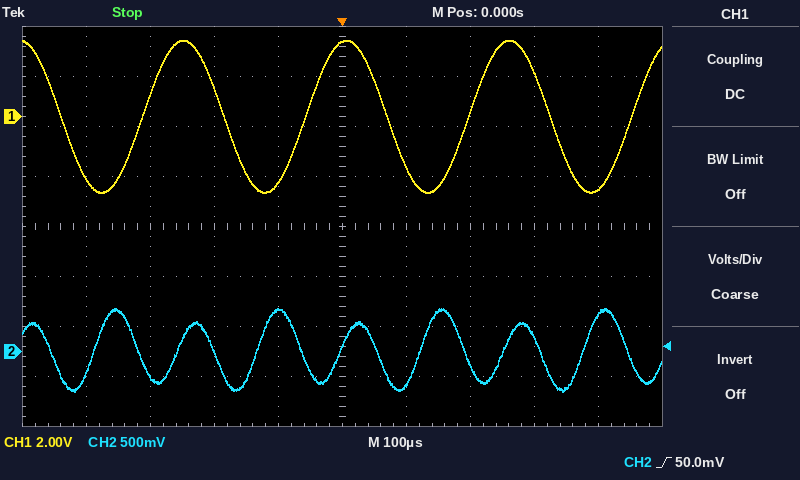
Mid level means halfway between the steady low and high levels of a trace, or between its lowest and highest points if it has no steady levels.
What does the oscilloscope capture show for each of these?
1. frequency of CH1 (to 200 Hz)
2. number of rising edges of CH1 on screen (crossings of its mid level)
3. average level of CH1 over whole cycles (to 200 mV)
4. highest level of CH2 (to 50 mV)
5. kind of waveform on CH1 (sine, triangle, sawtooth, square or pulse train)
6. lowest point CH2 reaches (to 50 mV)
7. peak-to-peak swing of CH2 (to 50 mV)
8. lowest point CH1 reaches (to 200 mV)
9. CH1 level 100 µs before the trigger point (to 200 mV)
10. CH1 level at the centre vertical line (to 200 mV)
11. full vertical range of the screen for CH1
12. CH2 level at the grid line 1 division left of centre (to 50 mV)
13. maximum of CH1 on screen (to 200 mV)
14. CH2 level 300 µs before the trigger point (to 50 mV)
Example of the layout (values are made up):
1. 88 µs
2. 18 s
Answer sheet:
1. 4.0 kHz
2. 4
3. 0.0 V
4. 450 mV
5. sine
6. -400 mV
7. 850 mV
8. -3.0 V
9. -2.6 V
10. 3.0 V
11. 16 V
12. 400 mV
13. 3.0 V
14. -250 mV
